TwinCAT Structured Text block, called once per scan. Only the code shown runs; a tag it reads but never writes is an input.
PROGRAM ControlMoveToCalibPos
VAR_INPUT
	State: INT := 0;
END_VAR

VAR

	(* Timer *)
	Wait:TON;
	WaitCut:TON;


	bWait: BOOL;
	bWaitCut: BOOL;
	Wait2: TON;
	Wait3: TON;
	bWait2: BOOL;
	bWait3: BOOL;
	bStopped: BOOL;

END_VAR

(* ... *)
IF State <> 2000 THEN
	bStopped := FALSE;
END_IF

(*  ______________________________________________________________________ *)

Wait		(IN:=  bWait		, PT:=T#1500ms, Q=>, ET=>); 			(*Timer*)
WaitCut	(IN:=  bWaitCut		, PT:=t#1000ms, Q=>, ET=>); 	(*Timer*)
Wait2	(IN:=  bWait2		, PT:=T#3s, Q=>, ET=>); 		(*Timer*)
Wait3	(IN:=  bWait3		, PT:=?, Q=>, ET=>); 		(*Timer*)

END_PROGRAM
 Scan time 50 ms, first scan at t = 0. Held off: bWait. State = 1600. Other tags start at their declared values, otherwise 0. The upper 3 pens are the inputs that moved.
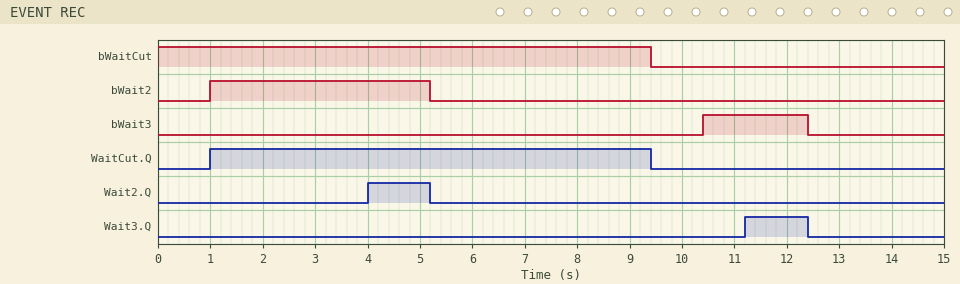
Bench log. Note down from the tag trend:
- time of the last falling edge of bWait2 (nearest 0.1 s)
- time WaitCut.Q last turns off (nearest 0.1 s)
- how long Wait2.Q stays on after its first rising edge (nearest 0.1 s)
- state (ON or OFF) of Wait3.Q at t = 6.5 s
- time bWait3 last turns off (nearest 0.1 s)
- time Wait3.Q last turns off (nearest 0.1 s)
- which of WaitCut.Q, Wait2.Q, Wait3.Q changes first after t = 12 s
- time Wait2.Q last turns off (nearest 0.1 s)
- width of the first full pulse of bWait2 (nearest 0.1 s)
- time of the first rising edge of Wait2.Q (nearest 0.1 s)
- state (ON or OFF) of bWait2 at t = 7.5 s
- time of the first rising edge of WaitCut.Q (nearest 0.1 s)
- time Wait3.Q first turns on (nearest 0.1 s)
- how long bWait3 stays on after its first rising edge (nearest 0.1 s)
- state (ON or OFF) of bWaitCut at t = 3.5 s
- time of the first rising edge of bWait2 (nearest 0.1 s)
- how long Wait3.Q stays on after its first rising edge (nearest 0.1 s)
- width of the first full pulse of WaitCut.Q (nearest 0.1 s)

5.2 s
9.4 s
1.2 s
OFF
12.4 s
12.4 s
Wait3.Q
5.2 s
4.2 s
4.0 s
OFF
1.0 s
11.2 s
2.0 s
ON
1.0 s
1.2 s
8.4 s
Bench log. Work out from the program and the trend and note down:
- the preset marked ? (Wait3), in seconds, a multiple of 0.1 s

0.8 s
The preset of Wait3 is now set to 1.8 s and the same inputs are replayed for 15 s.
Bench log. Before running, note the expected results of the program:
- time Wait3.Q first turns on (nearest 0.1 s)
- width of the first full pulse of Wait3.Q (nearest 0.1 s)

12.2 s
0.2 s
